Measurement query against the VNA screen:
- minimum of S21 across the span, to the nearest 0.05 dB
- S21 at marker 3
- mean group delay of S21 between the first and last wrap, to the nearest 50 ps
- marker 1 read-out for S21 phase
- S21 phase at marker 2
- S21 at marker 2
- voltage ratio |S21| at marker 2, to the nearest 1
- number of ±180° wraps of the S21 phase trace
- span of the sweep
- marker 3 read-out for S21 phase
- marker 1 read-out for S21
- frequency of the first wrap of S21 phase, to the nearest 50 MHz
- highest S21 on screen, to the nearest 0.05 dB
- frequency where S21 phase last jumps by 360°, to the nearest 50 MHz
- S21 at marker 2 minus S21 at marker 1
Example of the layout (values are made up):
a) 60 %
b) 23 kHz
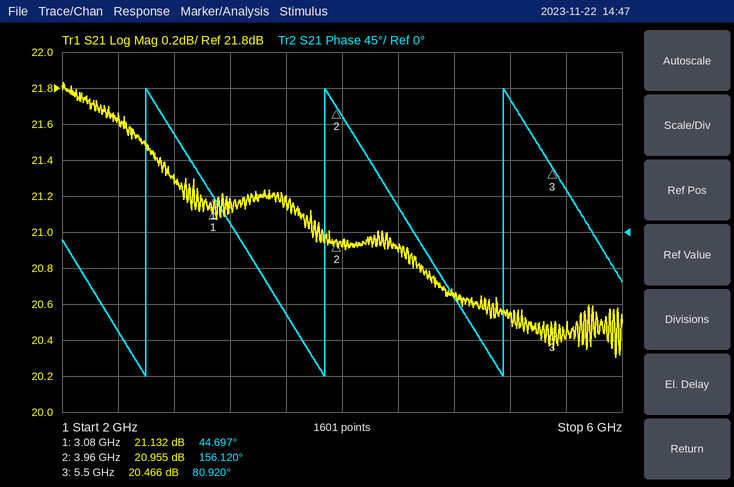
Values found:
a) 20.30 dB
b) 20.466 dB
c) 800 ps
d) 44.697°
e) 156.120°
f) 20.955 dB
g) 11
h) 3
i) 4 GHz
j) 80.920°
k) 21.132 dB
l) 2.60 GHz
m) 21.85 dB
n) 5.15 GHz
o) -0.177 dB
